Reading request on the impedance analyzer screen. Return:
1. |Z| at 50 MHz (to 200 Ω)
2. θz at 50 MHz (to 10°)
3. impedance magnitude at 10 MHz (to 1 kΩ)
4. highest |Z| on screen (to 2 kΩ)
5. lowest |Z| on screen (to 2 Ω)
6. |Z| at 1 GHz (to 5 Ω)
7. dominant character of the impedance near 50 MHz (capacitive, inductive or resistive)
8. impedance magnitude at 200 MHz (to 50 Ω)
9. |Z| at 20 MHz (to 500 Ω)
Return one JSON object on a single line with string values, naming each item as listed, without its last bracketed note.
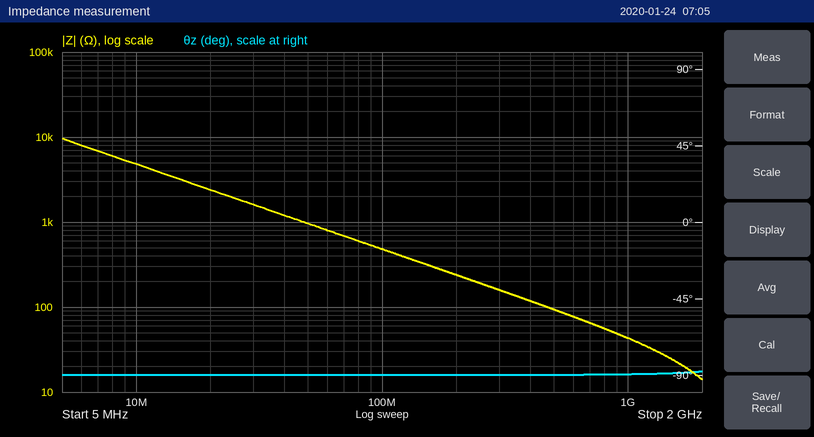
{"|Z| at 50 MHz": "1.0 kΩ", "θz at 50 MHz": "-90°", "impedance magnitude at 10 MHz": "5 kΩ", "highest |Z| on screen": "10 kΩ", "lowest |Z| on screen": "14 Ω", "|Z| at 1 GHz": "45 Ω", "dominant character of the impedance near 50 MHz": "capacitive", "impedance magnitude at 200 MHz": "250 Ω", "|Z| at 20 MHz": "2.5 kΩ"}
